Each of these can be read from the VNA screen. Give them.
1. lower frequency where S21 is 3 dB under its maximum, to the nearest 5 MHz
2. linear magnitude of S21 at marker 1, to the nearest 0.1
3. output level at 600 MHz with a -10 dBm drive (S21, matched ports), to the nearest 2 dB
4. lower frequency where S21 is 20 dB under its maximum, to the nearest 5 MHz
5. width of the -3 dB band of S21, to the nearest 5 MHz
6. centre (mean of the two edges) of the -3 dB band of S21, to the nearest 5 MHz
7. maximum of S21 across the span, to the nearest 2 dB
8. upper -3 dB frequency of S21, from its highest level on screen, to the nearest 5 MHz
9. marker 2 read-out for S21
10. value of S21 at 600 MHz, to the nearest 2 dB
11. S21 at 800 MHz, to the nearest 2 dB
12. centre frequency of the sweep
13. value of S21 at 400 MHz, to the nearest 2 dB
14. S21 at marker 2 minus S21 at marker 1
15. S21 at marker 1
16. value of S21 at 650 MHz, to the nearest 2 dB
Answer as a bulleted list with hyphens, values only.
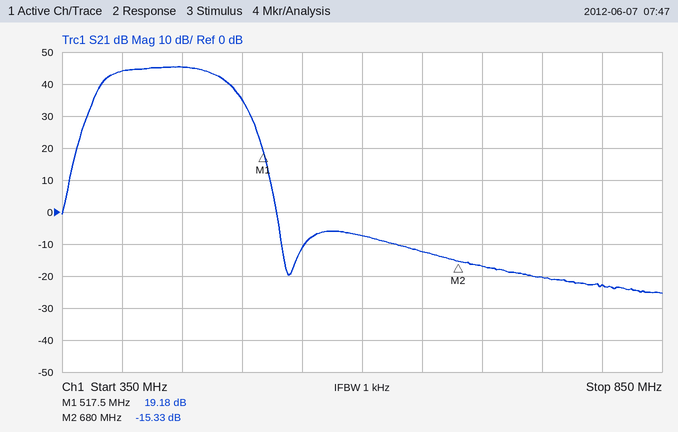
- 390 MHz
- 9.1
- -18 dBm
- 365 MHz
- 90 MHz
- 435 MHz
- 46 dB
- 480 MHz
- -15.33 dB
- -8 dB
- -22 dB
- 600 MHz
- 44 dB
- -34.51 dB
- 19.18 dB
- -12 dB
